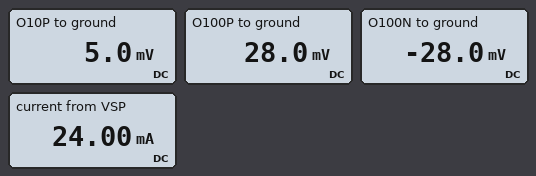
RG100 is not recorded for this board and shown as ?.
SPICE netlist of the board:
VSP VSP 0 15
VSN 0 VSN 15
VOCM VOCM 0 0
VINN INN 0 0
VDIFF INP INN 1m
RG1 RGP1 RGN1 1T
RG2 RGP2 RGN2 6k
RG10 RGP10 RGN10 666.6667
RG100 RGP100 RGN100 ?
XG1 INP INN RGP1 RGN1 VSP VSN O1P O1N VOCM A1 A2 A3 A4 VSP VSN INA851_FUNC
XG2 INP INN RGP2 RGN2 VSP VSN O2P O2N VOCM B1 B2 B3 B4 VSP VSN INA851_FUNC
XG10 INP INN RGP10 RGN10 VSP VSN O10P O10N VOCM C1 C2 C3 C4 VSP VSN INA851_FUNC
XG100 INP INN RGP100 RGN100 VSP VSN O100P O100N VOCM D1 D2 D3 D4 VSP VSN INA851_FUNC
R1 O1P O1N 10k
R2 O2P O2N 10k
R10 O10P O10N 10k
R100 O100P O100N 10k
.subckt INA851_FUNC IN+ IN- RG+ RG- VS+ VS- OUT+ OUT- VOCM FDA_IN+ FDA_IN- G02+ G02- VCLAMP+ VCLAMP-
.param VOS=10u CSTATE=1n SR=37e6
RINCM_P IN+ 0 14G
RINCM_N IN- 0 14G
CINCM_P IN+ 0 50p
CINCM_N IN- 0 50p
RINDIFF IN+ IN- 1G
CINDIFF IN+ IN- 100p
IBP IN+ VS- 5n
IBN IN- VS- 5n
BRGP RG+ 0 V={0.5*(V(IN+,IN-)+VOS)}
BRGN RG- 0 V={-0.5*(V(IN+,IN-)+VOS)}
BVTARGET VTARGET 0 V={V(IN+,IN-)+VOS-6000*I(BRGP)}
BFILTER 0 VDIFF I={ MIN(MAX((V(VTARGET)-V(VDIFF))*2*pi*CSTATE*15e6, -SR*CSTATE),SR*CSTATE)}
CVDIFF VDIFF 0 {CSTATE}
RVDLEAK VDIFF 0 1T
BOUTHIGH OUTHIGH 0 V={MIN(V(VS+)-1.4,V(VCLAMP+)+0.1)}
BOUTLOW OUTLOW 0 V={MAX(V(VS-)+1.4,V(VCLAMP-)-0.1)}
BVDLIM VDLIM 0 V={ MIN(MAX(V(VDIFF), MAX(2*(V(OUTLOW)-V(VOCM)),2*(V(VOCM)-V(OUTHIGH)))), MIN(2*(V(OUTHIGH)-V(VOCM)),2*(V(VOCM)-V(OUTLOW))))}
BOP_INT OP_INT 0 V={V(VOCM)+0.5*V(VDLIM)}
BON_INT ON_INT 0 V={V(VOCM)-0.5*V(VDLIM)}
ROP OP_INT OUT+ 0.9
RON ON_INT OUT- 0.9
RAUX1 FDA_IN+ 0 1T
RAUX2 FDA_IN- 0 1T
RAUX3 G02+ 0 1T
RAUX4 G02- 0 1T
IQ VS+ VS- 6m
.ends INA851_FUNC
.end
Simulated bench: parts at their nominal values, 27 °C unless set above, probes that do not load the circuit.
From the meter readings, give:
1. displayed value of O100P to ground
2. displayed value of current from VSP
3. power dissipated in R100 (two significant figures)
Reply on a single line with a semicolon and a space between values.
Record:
28.0 mV; 24.00 mA; 310 nW
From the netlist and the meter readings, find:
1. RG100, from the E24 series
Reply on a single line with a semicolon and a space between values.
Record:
110 Ω
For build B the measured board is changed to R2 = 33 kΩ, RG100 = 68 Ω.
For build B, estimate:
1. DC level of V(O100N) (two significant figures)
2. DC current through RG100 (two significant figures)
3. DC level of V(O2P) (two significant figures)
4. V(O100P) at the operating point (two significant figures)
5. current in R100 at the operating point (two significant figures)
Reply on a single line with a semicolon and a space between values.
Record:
-45 mV; 15 µA; 1.0 mV; 45 mV; 9.0 µA
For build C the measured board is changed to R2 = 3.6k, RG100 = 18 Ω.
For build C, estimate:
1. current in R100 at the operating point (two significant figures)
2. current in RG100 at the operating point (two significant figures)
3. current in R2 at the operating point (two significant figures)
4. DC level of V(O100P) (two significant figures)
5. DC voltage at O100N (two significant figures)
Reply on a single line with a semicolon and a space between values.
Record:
34 µA; 56 µA; 560 nA; 170 mV; -170 mV
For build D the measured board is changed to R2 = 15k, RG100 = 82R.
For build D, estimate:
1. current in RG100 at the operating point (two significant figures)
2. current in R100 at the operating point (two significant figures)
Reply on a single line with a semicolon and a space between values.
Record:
12 µA; 7.5 µA
